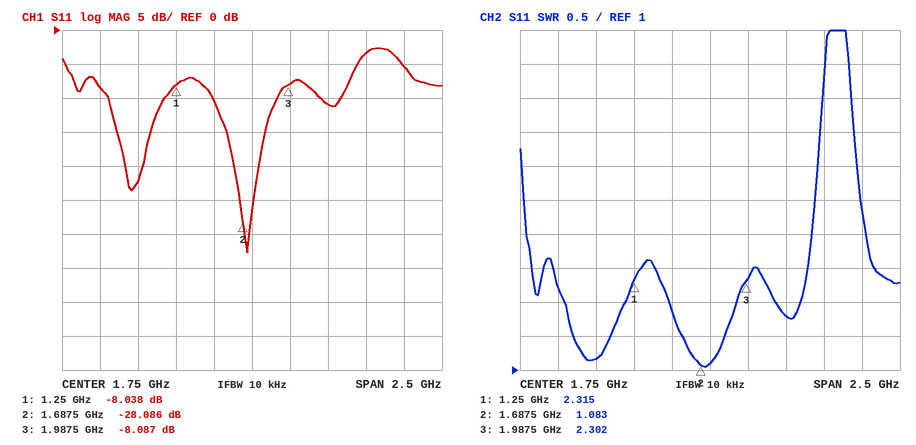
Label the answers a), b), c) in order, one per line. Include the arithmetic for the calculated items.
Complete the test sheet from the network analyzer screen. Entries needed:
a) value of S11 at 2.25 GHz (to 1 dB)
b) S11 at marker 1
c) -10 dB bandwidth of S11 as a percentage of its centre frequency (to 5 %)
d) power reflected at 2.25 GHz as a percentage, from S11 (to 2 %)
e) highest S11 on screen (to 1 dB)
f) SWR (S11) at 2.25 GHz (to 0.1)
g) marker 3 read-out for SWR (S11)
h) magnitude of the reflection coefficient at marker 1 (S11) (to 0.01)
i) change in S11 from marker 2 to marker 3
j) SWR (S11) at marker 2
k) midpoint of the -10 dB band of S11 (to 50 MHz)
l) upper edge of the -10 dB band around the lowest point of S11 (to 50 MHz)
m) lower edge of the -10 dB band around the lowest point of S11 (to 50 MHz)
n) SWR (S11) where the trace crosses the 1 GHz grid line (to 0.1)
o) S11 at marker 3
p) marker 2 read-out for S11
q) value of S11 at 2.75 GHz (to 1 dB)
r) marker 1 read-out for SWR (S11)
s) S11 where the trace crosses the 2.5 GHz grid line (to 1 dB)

a) -11 dB
b) -8.038 dB
c) 400 MHz / 1.7 GHz ≈ 23.5 %, so 25 % to the nearest 5 %
d) 10^(-11/10) ≈ 8 %
e) -3 dB
f) 1.8
g) 2.302
h) 10^(-8.038/20) ≈ 0.40
i) -8.087 − (-28.086) = 19.999 dB
j) 1.083
k) 1.70 GHz
l) 1.90 GHz
m) 1.50 GHz
n) 1.2
o) -8.087 dB
p) -28.086 dB
q) -5 dB
r) 2.315
s) -3 dB
